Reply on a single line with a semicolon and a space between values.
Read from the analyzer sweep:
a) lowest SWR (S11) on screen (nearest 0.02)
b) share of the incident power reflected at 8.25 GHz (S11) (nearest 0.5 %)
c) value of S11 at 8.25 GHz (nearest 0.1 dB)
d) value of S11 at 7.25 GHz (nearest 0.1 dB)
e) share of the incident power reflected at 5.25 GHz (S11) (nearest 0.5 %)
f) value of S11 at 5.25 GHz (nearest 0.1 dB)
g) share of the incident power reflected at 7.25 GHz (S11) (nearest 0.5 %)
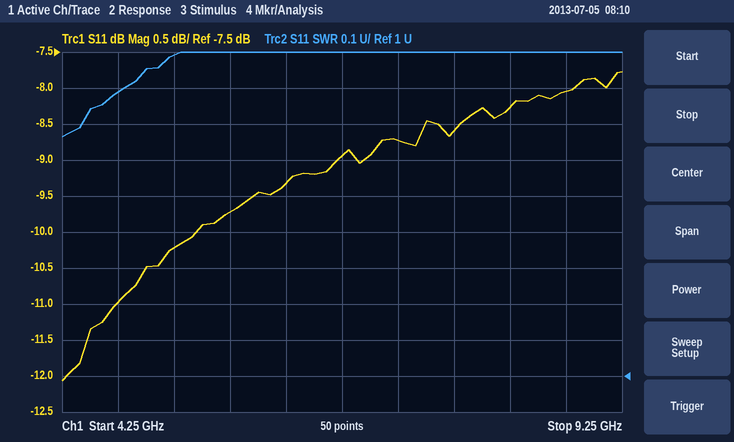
1.66; 15.0 %; -8.3 dB; -8.7 dB; 9.5 %; -10.2 dB; 13.5 %
